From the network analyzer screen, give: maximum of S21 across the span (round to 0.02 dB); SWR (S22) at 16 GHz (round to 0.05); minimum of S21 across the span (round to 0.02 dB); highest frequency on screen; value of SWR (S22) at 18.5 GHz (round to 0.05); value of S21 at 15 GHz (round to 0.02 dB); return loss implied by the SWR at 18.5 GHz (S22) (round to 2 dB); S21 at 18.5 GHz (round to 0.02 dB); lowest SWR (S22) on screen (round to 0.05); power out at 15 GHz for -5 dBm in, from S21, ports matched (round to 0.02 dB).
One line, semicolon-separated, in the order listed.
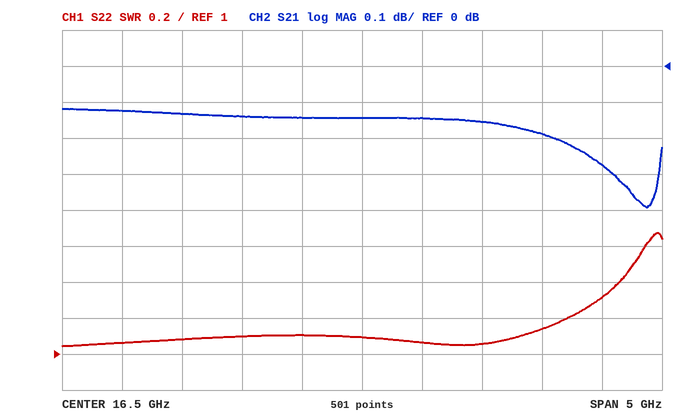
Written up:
-0.12 dB; 1.10; -0.40 dB; 19 GHz; 1.30; -0.14 dB; 18 dB; -0.28 dB; 1.05; -5.14 dBm
